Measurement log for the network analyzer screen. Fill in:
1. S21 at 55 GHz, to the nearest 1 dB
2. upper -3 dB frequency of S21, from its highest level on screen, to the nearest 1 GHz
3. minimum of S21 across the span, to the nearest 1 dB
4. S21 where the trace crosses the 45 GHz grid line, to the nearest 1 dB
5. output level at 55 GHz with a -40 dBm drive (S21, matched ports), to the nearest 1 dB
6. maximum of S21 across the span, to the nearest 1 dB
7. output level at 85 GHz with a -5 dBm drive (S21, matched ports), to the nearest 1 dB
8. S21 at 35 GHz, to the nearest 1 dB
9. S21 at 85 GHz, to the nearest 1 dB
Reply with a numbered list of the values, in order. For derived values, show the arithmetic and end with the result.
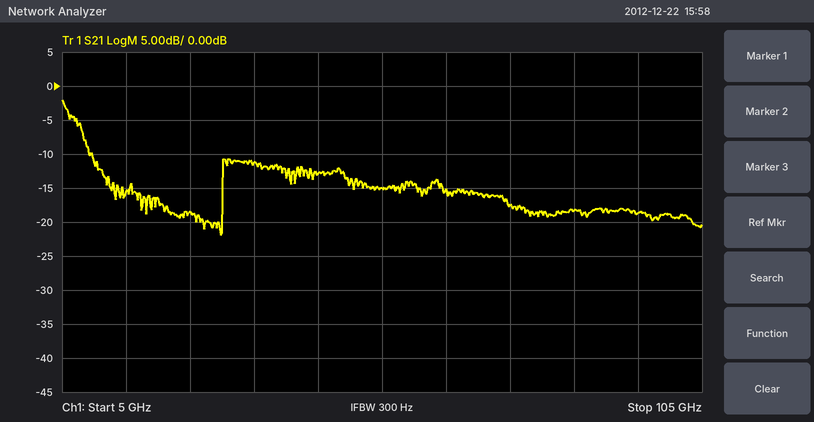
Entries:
1. -15 dB
2. 7 GHz
3. -22 dB
4. -13 dB
5. -40 dBm + (-15 dB) = -55 dBm
6. -2 dB
7. -5 dBm + (-18 dB) = -23 dBm
8. -11 dB
9. -18 dB
